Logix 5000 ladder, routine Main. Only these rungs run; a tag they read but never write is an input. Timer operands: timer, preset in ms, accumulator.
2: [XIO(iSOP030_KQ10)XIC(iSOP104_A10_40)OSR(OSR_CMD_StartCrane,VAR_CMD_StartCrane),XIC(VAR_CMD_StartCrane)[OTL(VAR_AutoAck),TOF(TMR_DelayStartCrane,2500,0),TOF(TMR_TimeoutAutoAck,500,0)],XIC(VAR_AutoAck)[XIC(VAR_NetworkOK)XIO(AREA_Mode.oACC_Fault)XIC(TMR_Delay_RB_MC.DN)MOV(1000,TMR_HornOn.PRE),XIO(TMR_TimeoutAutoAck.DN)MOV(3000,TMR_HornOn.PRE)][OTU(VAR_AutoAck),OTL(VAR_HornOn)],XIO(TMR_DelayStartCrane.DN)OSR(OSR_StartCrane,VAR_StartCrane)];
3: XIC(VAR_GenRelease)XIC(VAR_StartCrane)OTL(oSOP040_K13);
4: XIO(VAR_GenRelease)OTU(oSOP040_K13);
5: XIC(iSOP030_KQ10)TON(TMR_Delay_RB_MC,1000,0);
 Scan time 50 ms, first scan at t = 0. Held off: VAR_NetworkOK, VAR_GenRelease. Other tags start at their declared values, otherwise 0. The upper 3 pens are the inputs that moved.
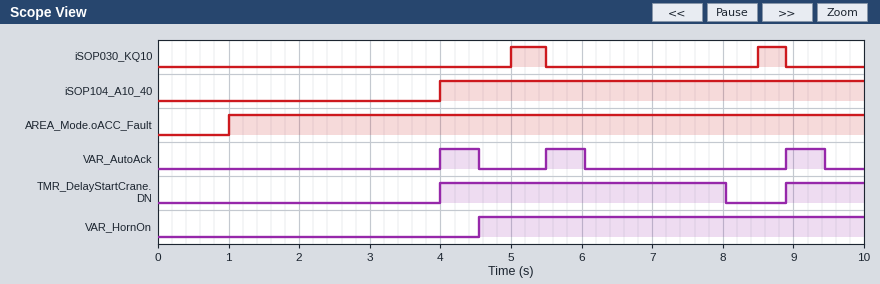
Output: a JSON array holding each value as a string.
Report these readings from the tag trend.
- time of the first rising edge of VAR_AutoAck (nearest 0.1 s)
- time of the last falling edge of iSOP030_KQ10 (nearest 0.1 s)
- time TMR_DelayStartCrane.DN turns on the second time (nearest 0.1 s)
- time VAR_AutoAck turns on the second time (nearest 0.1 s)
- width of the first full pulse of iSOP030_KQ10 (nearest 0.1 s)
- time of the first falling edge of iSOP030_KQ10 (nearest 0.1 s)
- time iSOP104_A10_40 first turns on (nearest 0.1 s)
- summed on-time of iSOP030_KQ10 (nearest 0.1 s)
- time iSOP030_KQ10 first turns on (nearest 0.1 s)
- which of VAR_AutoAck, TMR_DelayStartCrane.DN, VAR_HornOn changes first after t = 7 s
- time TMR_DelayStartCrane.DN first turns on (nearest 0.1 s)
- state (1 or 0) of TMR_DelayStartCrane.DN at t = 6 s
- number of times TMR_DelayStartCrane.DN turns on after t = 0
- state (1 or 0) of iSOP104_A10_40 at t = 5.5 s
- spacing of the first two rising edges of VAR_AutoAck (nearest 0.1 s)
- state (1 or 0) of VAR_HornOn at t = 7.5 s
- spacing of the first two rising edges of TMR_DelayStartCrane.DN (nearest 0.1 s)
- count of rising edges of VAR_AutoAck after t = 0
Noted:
["4.0 s", "8.9 s", "8.9 s", "5.5 s", "0.5 s", "5.5 s", "4.0 s", "0.9 s", "5.0 s", "TMR_DelayStartCrane.DN", "4.0 s", "1", "2", "1", "1.5 s", "1", "4.9 s", "3"]
